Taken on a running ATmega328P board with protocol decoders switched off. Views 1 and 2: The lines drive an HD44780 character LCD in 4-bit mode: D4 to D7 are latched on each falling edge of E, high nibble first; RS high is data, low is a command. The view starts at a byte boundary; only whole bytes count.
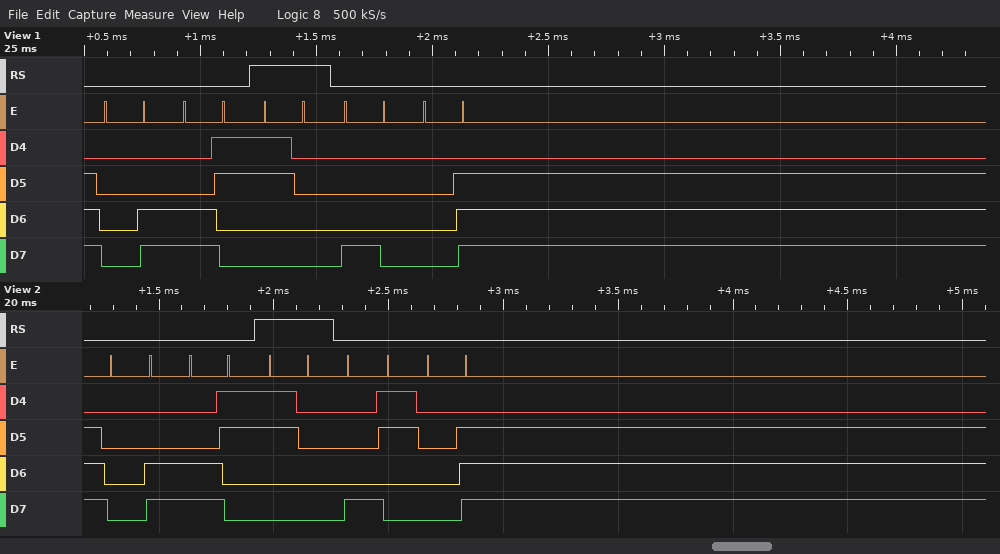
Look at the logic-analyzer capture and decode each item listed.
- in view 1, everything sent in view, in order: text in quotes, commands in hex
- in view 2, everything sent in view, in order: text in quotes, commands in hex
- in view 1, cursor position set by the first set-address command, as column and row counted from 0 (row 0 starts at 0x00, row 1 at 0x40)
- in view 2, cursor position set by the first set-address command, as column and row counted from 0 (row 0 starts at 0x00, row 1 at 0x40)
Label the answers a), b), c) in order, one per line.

a) 0x0C 0xC3 "0" 0x80 0x0E
b) 0x0C 0xC3 "0" 0x83 0x0E
c) column 3, row 1
d) column 3, row 1
